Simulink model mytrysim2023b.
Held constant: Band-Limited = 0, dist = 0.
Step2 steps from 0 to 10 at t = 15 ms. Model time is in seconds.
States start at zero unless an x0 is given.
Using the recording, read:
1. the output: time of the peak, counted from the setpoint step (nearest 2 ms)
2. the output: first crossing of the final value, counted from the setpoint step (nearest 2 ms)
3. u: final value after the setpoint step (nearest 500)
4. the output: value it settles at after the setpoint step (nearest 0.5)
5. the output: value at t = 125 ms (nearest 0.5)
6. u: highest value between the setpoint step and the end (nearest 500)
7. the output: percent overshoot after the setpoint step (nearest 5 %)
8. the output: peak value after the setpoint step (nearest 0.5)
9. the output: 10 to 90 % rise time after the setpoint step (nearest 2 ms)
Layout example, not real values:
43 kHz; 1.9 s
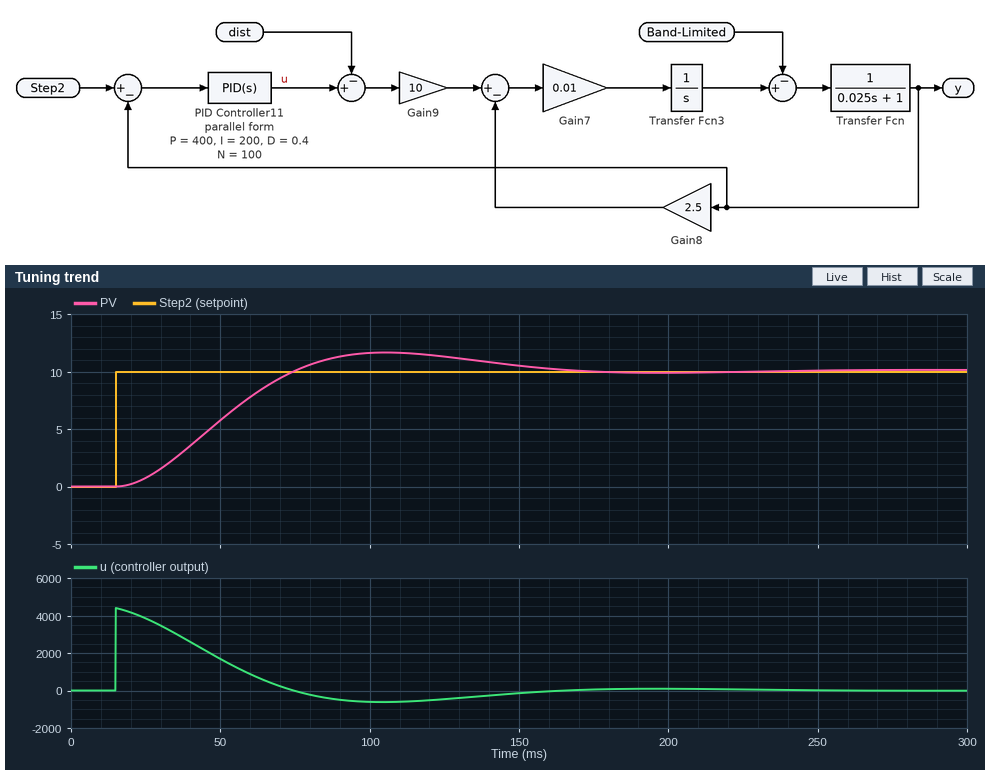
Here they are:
90 ms; 60 ms; 0; 10.0; 11.5; 4500; 15 %; 11.5; 40 ms
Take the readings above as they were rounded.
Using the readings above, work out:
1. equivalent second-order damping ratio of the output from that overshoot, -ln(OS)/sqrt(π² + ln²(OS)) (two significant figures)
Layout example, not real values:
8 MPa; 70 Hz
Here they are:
0.52
